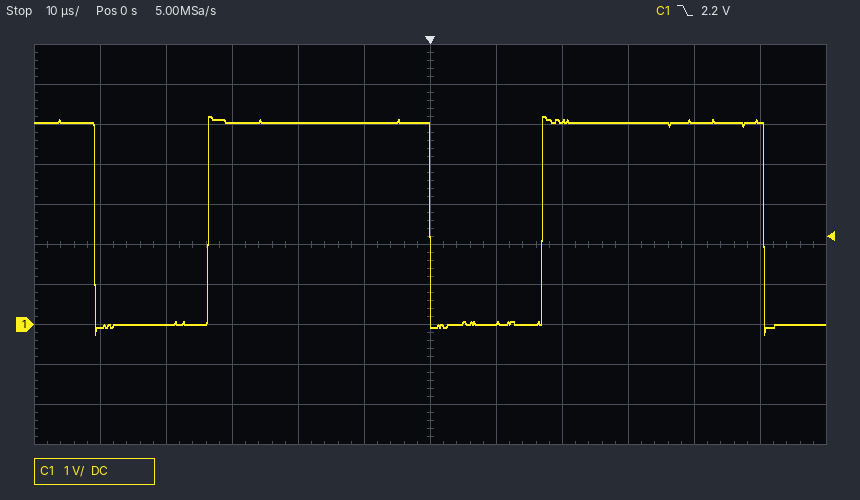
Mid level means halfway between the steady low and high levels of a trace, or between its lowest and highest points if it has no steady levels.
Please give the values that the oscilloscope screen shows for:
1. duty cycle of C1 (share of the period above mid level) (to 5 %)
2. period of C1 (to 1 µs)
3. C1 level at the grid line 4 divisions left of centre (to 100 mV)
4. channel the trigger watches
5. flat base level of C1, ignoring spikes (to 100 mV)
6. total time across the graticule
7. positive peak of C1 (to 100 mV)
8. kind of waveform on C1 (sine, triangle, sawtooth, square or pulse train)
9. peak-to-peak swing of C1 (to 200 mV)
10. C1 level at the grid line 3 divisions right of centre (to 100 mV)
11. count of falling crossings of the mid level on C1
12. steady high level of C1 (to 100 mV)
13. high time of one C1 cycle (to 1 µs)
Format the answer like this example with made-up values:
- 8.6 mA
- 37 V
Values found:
- 65 %
- 51 µs
- 0.0 V
- C1
- 0.0 V
- 120 µs
- 5.2 V
- pulse train
- 5.4 V
- 5.0 V
- 3
- 5.0 V
- 34 µs
